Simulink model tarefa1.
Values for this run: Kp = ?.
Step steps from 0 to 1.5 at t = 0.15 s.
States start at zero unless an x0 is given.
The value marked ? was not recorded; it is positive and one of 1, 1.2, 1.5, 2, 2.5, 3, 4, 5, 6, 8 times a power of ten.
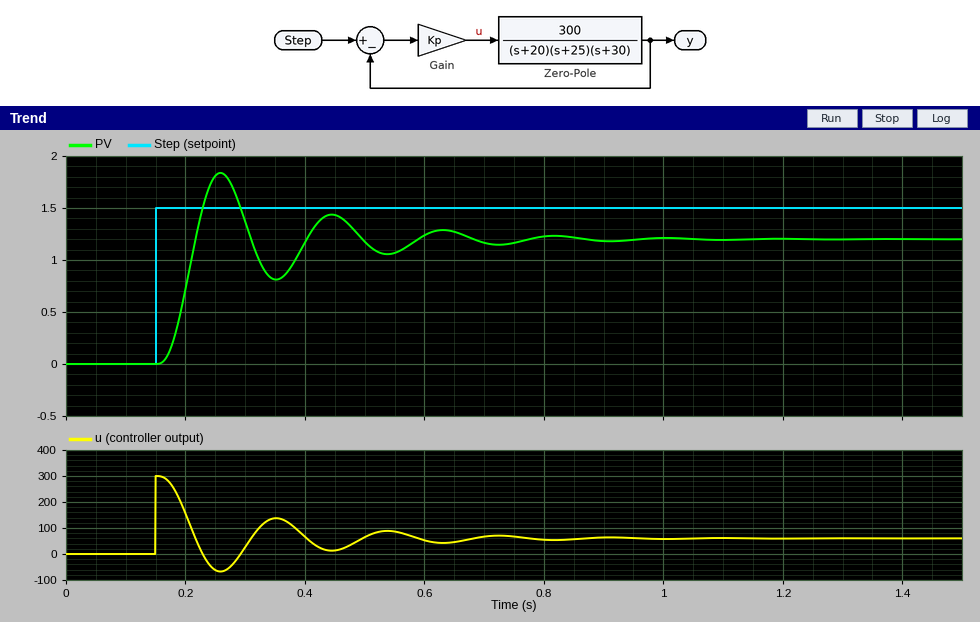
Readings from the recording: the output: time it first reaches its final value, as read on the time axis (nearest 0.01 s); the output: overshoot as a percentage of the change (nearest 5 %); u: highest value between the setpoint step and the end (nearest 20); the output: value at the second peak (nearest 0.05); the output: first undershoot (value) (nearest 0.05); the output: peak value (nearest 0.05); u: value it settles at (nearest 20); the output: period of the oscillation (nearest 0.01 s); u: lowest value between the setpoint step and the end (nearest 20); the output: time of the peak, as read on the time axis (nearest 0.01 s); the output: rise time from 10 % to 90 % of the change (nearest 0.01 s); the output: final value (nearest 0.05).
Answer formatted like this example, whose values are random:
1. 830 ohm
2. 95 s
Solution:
1. 0.22 s
2. 55 %
3. 300
4. 1.45
5. 0.80
6. 1.85
7. 60
8. 0.19 s
9. -60
10. 0.26 s
11. 0.04 s
12. 1.20
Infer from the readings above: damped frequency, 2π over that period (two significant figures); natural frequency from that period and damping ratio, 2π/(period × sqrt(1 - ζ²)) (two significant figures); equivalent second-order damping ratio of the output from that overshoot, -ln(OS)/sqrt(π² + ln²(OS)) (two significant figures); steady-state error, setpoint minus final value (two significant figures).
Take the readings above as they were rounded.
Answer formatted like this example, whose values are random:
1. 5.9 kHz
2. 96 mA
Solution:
1. 33 rad/s
2. 34 rad/s
3. 0.19
4. 0.30
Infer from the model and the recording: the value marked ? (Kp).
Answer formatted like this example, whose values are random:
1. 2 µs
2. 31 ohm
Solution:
1. 200
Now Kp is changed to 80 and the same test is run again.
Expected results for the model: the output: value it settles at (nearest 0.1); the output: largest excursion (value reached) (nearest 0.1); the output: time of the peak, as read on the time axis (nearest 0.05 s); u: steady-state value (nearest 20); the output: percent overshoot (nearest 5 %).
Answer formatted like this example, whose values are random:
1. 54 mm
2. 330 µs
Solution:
1. 0.9
2. 1.1
3. 0.30 s
4. 40
5. 25 %
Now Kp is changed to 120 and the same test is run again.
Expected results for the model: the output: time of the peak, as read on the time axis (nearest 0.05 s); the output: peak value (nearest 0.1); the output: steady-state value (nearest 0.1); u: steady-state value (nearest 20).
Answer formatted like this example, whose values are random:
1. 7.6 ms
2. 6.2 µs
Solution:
1. 0.30 s
2. 1.4
3. 1.1
4. 60
